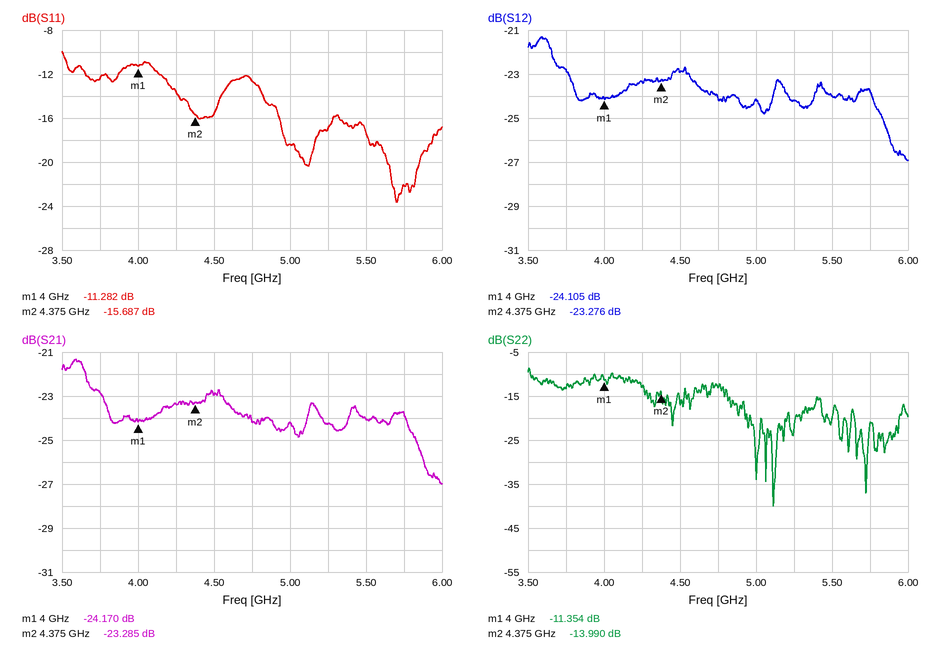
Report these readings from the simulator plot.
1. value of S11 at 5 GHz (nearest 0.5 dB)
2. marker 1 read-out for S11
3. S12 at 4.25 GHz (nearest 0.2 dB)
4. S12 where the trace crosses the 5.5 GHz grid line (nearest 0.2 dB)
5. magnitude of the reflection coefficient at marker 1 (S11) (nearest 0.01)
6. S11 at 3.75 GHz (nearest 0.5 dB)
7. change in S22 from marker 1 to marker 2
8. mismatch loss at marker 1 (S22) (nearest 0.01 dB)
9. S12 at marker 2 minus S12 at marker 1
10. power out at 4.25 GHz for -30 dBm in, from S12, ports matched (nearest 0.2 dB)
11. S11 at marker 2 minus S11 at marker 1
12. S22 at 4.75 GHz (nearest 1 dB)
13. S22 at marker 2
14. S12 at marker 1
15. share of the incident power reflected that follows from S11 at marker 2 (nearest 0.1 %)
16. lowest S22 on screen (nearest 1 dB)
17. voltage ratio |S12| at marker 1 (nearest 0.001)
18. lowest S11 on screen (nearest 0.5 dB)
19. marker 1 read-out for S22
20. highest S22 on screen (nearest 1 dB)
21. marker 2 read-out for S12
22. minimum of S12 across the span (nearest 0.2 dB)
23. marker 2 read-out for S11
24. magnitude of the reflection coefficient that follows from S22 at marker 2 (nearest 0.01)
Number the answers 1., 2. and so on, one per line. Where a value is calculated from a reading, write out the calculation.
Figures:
1. -18.5 dB
2. -11.282 dB
3. -23.4 dB
4. -24.0 dB
5. 10^(-11.282/20) ≈ 0.27
6. -12.5 dB
7. -13.99 − (-11.354) = -2.636 dB
8. −10 log10(1 − 10^(-11.354/10)) ≈ 0.33 dB
9. -23.276 − (-24.105) = 0.829 dB
10. -30 dBm + (-23.4 dB) = -53.4 dBm
11. -15.687 − (-11.282) = -4.405 dB
12. -13 dB
13. -13.990 dB
14. -24.105 dB
15. 10^(-15.687/10) ≈ 2.7 %
16. -40 dB
17. 10^(-24.105/20) ≈ 0.062
18. -23.5 dB
19. -11.354 dB
20. -9 dB
21. -23.276 dB
22. -27.0 dB
23. -15.687 dB
24. 10^(-13.99/20) ≈ 0.20
